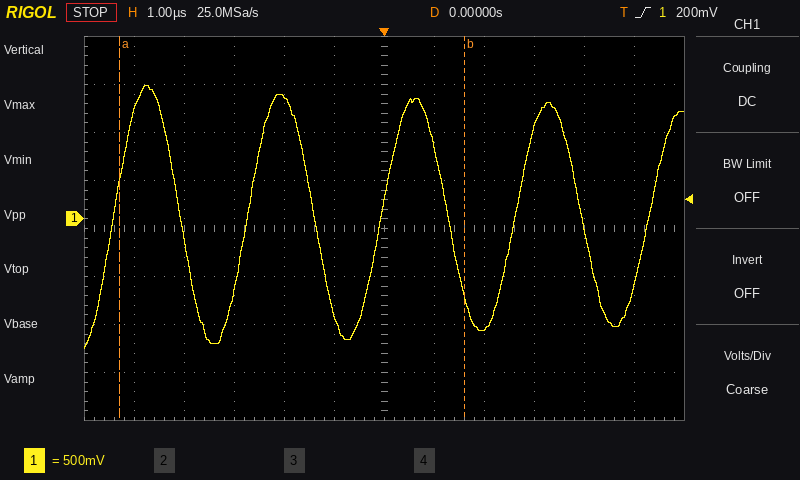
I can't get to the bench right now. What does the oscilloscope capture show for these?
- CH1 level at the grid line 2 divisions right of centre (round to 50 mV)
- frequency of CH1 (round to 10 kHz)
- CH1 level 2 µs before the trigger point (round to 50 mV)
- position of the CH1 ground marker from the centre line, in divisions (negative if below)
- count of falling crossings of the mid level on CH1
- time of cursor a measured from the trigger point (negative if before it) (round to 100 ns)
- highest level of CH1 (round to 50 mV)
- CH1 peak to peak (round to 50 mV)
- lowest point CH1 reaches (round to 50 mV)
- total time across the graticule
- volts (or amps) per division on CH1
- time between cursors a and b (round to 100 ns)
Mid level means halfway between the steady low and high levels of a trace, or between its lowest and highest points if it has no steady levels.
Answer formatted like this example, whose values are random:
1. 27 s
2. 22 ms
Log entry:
1. -1.15 V
2. 370 kHz
3. 1.25 V
4. +0.2 div
5. 4
6. -5.3 µs
7. 1.40 V
8. 2.75 V
9. -1.35 V
10. 12 µs
11. 500 mV
12. 6.9 µs
